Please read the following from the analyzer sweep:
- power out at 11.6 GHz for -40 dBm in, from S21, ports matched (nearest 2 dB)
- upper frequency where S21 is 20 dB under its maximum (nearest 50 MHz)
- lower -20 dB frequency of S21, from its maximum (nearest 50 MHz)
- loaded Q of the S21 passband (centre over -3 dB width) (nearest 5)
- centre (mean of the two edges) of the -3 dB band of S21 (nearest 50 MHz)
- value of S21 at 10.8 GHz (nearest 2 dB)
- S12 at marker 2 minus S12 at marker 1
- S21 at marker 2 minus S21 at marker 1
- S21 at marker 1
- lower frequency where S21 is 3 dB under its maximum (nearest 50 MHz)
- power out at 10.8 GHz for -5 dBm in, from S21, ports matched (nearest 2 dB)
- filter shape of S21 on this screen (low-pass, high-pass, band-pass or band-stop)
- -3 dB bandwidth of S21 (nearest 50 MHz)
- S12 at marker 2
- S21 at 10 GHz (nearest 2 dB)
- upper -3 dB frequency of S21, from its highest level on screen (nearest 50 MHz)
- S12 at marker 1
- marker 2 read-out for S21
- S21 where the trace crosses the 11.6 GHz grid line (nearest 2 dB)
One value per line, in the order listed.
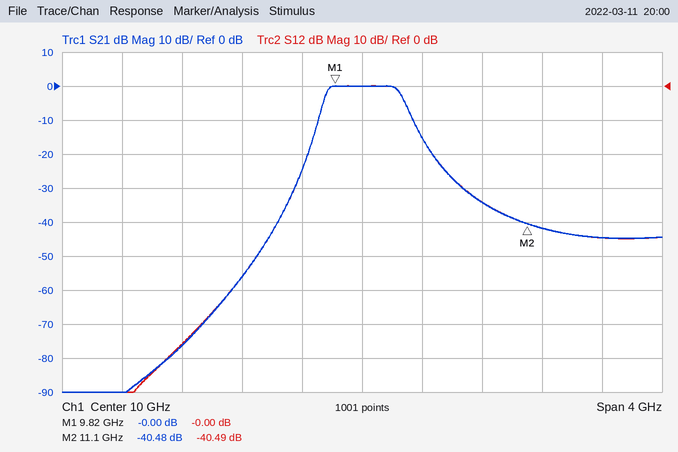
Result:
-84 dBm
10.45 GHz
9.65 GHz
20
10.00 GHz
-34 dB
-40.49 dB
-40.48 dB
-0.00 dB
9.75 GHz
-40 dBm
band-pass
500 MHz
-40.49 dB
0 dB
10.25 GHz
-0.00 dB
-40.48 dB
-44 dB
